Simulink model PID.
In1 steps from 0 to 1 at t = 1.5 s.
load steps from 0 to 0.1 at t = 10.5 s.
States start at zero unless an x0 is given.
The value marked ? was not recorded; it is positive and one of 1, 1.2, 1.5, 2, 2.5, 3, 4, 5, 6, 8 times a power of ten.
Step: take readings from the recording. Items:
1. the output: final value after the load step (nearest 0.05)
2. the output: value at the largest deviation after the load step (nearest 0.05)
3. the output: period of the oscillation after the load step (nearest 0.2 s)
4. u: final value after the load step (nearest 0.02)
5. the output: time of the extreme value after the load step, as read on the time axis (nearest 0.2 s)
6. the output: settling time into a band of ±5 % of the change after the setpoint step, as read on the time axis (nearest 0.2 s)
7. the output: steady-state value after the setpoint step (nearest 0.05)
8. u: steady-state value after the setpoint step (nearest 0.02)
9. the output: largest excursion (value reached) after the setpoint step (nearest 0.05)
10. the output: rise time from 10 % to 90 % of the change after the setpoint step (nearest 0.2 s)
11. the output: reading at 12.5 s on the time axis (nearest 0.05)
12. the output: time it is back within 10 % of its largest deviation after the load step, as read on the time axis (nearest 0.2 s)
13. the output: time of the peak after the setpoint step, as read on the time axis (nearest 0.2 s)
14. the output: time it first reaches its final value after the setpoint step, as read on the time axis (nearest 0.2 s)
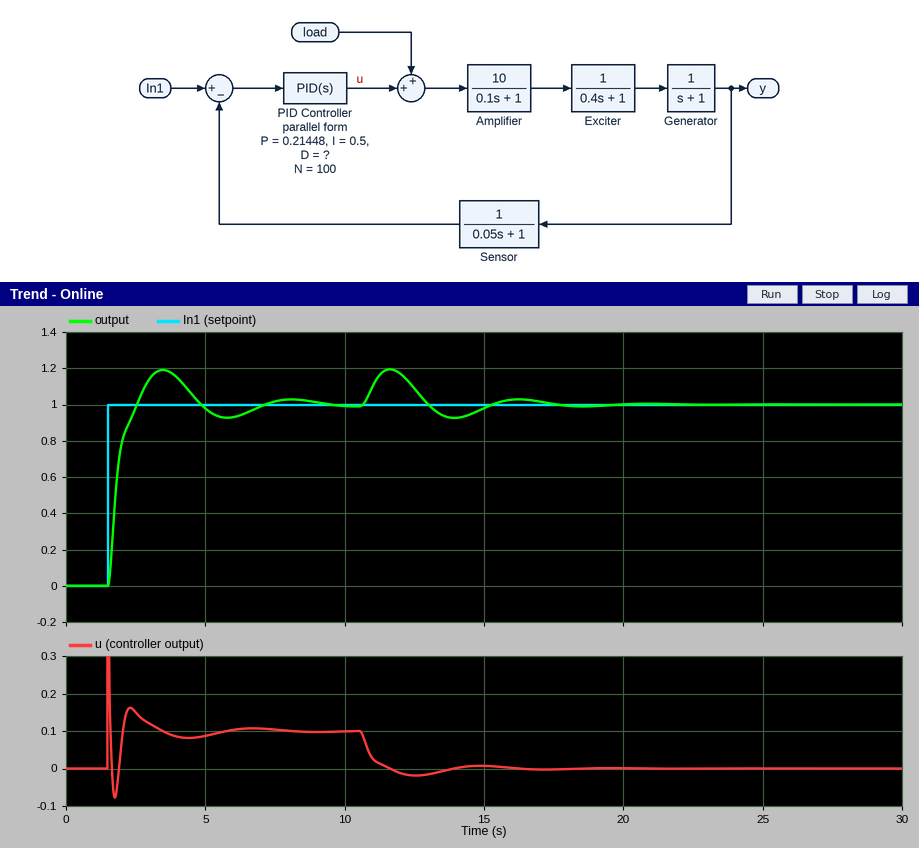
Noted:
1.00
1.20
4.6 s
0.00
11.6 s
6.4 s
1.00
0.10
1.20
0.6 s
1.10
16.8 s
3.4 s
2.6 s
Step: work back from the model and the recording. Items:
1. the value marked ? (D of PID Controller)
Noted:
0.15
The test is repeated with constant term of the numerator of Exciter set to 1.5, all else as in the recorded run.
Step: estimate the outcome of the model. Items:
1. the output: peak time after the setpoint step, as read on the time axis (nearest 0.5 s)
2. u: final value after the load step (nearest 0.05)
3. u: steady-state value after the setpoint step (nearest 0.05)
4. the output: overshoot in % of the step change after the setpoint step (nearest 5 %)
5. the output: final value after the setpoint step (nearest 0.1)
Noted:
3.0 s
-0.05
0.05
15 %
1.0
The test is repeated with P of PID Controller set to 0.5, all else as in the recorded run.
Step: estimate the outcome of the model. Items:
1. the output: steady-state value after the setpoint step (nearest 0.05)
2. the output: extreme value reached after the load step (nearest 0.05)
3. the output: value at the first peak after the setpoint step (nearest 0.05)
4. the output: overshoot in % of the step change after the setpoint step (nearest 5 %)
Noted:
1.00
1.15
1.10
10 %
